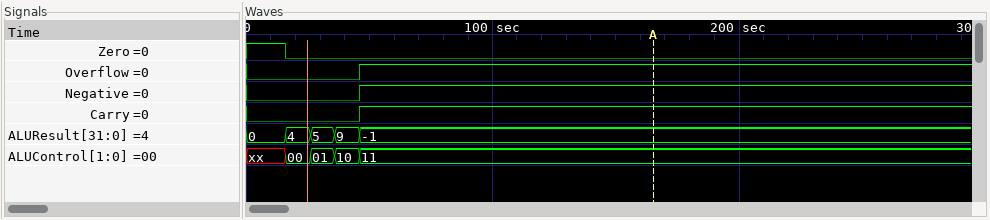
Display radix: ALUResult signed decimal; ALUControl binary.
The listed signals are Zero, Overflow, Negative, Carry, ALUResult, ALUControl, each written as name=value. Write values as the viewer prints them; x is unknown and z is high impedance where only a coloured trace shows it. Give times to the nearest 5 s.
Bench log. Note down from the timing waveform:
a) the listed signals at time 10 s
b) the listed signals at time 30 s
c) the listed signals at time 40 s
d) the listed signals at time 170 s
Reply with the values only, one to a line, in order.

Zero=1, Overflow=0, Negative=0, Carry=0, ALUResult=0, ALUControl=xx
Zero=0, Overflow=0, Negative=0, Carry=0, ALUResult=5, ALUControl=01
Zero=0, Overflow=0, Negative=0, Carry=0, ALUResult=9, ALUControl=10
Zero=0, Overflow=1, Negative=1, Carry=1, ALUResult=-1, ALUControl=11
